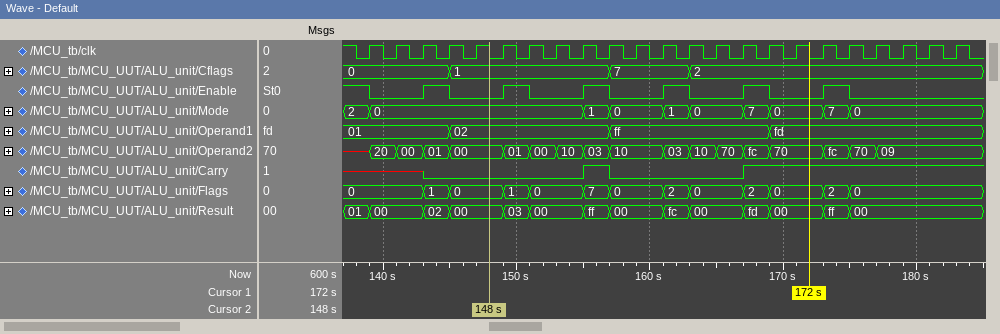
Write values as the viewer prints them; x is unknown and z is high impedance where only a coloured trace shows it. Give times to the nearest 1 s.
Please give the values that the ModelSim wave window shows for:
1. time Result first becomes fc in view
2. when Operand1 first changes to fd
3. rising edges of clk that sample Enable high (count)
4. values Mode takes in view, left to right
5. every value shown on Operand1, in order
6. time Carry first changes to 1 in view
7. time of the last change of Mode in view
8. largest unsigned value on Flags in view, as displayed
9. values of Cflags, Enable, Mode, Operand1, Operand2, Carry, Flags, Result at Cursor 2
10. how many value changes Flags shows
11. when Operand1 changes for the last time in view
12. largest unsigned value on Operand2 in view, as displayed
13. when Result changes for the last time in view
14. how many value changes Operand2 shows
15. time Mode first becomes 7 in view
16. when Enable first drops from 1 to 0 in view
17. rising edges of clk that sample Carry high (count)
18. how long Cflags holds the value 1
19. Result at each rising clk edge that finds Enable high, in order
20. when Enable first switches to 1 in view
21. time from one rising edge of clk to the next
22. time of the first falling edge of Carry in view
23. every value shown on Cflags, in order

161 s
169 s
7
2, 0, 1, 0, 1, 0, 7, 0, 7, 0
01, 02, ff, fd
155 s
175 s
7
Cflags=1, Enable=0, Mode=0, Operand1=02, Operand2=00, Carry=0, Flags=0, Result=00
12
169 s
fc
175 s
17
167 s
139 s
9
12 s
01, 02, 03, ff, fc, fd, ff
143 s
2 s
157 s
0, 1, 7, 2
